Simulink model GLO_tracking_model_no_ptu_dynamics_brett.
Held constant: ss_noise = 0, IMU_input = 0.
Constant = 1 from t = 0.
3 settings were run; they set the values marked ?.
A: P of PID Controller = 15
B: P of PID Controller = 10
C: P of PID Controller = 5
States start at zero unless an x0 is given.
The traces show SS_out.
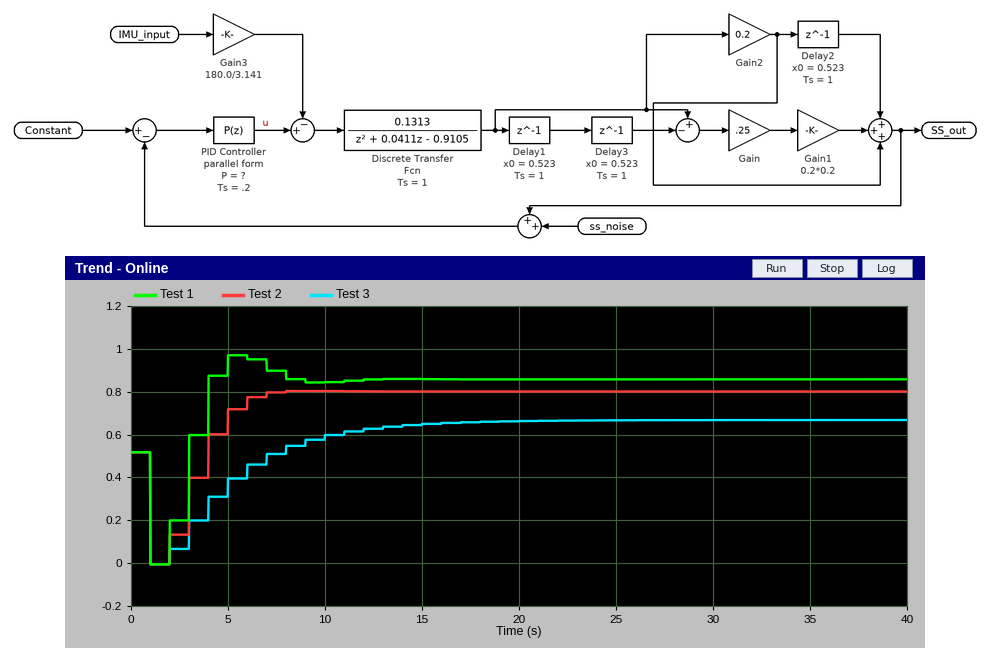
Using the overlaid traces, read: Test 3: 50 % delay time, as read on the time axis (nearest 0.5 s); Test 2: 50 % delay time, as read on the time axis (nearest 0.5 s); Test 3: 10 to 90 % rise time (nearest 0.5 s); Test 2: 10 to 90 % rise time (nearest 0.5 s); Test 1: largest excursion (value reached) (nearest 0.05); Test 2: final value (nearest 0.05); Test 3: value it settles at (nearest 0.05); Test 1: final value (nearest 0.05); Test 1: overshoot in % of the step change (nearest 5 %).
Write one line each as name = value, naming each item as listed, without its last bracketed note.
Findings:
Test 3: 50 % delay time, as read on the time axis = 10.0 s
Test 2: 50 % delay time, as read on the time axis = 5.0 s
Test 3: 10 to 90 % rise time = 8.0 s
Test 2: 10 to 90 % rise time = 2.0 s
Test 1: largest excursion (value reached) = 0.95
Test 2: final value = 0.80
Test 3: value it settles at = 0.65
Test 1: final value = 0.85
Test 1: overshoot in % of the step change = 35 %
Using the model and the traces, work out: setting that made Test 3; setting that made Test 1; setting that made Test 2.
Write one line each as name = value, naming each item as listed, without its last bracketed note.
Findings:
setting that made Test 3 = C
setting that made Test 1 = A
setting that made Test 2 = B
